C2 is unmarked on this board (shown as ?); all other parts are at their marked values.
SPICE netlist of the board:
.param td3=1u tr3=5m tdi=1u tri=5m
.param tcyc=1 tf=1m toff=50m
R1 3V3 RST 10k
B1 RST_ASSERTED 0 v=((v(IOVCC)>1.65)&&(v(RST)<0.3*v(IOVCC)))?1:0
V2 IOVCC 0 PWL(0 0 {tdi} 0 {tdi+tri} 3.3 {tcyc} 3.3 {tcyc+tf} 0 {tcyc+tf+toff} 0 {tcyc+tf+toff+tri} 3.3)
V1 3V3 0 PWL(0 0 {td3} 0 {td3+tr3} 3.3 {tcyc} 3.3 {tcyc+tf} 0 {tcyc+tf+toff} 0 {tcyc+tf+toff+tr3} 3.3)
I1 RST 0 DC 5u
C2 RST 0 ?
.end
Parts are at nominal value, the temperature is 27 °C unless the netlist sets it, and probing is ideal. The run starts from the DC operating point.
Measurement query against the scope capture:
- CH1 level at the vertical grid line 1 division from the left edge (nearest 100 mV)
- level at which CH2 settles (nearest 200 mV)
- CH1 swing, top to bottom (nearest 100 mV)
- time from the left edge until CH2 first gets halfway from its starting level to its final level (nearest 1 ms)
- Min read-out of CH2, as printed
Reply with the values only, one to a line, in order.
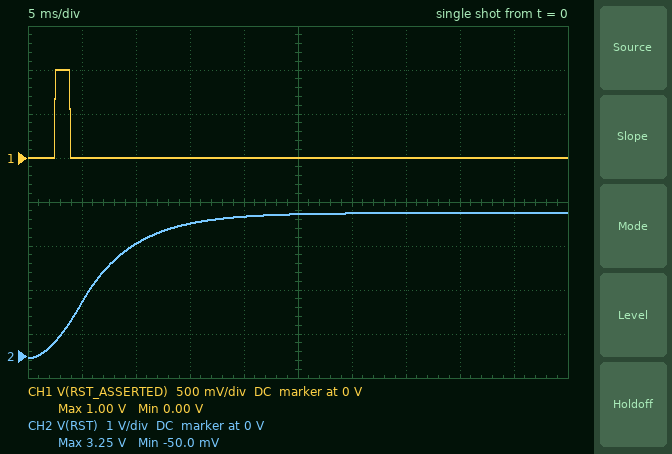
0 V
3.2 V
1.0 V
6 ms
-50.0 mV
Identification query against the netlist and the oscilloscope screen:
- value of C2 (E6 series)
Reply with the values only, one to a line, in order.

470 nF
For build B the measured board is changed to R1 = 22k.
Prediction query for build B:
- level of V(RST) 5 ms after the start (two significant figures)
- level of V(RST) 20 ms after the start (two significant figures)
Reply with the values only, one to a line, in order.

570 mV
2.6 V
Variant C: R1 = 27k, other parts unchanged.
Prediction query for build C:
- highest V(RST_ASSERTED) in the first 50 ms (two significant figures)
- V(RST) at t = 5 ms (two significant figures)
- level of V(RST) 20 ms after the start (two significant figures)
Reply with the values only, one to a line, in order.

1.0 V
440 mV
2.3 V
